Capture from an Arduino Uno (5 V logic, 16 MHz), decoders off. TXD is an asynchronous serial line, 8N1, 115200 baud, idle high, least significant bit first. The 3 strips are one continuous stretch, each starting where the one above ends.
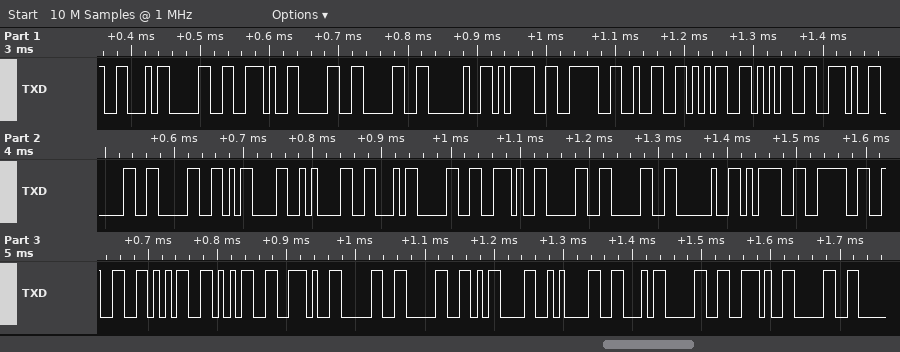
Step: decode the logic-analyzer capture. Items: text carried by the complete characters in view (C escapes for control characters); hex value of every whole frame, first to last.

"F0.00 =>255.00\r\nF0.00 =>255.00\r\nF0.0"
46 30 2E 30 30 20 3D 3E 32 35 35 2E 30 30 0D 0A 46 30 2E 30 30 20 3D 3E 32 35 35 2E 30 30 0D 0A 46 30 2E 30
